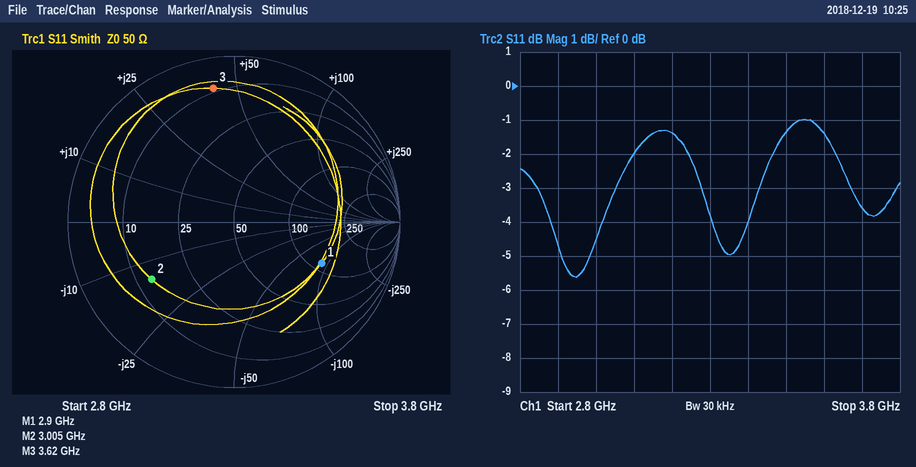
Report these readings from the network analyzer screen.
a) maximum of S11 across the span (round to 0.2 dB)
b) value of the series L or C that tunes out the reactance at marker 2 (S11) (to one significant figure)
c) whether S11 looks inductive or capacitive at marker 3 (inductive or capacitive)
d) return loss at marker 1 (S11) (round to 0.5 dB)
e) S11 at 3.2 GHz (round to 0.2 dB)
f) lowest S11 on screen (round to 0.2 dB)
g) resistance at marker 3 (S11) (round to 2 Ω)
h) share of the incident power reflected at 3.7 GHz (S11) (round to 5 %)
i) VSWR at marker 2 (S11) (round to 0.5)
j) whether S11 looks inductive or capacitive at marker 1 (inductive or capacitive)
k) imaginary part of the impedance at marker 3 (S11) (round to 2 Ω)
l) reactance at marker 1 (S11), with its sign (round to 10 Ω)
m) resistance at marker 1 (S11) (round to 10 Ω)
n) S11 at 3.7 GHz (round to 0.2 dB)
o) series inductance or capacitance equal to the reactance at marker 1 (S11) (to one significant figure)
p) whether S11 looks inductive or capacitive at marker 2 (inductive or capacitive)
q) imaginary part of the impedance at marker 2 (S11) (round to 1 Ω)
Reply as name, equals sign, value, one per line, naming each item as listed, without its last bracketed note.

maximum of S11 across the span = -1.0 dB
value of the series L or C that tunes out the reactance at marker 2 (S11) = 800 pH
whether S11 looks inductive or capacitive at marker 3 = inductive
return loss at marker 1 (S11) = 4.5 dB
S11 at 3.2 GHz = -1.4 dB
lowest S11 on screen = -5.6 dB
resistance at marker 3 (S11) = 8 Ω
share of the incident power reflected at 3.7 GHz (S11) = 45 %
VSWR at marker 2 (S11) = 4.0
whether S11 looks inductive or capacitive at marker 1 = capacitive
imaginary part of the impedance at marker 3 (S11) = +42 Ω
reactance at marker 1 (S11), with its sign = -90 Ω
resistance at marker 1 (S11) = 120 Ω
S11 at 3.7 GHz = -3.6 dB
series inductance or capacitance equal to the reactance at marker 1 (S11) = 600 fF
whether S11 looks inductive or capacitive at marker 2 = capacitive
imaginary part of the impedance at marker 2 (S11) = -15 Ω
